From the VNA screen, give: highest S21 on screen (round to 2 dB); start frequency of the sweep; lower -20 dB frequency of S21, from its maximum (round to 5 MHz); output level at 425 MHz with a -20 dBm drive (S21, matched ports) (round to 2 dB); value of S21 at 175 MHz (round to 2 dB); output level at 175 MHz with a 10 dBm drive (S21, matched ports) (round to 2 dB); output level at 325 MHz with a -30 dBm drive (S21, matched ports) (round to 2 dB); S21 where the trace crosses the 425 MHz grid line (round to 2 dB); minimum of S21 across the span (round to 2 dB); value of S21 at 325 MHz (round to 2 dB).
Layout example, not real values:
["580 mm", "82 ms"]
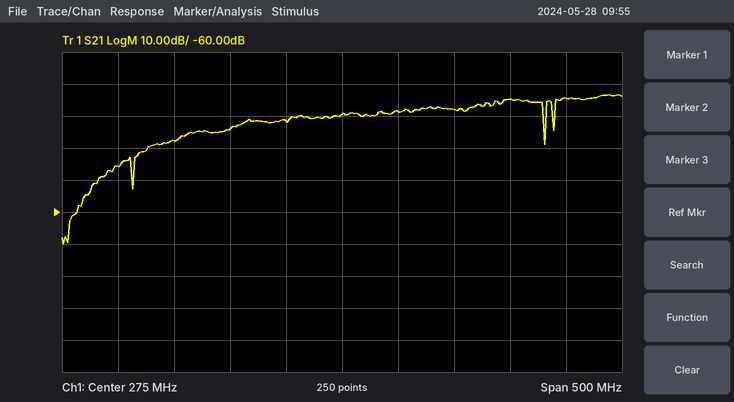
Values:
["-24 dB", "25 MHz", "90 MHz", "-44 dBm", "-34 dB", "-24 dBm", "-58 dBm", "-24 dB", "-70 dB", "-28 dB"]
